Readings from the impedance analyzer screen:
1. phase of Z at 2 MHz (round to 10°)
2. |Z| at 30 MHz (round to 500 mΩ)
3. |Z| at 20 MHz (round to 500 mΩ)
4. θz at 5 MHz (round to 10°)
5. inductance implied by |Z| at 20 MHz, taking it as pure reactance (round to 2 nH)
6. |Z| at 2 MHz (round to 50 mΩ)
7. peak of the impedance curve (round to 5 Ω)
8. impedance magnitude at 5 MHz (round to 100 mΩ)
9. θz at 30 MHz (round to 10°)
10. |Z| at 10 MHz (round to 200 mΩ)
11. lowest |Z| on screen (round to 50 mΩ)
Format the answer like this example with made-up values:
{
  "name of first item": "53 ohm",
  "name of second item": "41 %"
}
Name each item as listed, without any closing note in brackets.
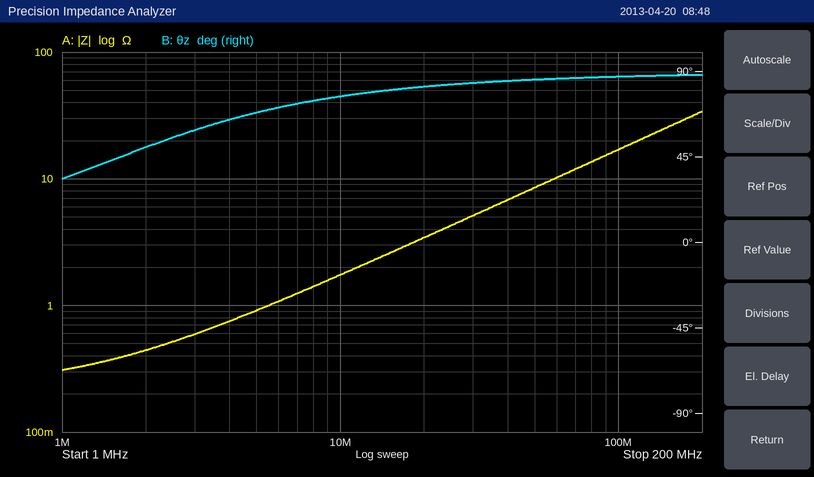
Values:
{
  "phase of Z at 2 MHz": "50°",
  "|Z| at 30 MHz": "5.0 Ω",
  "|Z| at 20 MHz": "3.5 Ω",
  "θz at 5 MHz": "70°",
  "inductance implied by |Z| at 20 MHz, taking it as pure reactance": "28 nH",
  "|Z| at 2 MHz": "450 mΩ",
  "peak of the impedance curve": "35 Ω",
  "impedance magnitude at 5 MHz": "900 mΩ",
  "θz at 30 MHz": "80°",
  "|Z| at 10 MHz": "1.8 Ω",
  "lowest |Z| on screen": "300 mΩ"
}
